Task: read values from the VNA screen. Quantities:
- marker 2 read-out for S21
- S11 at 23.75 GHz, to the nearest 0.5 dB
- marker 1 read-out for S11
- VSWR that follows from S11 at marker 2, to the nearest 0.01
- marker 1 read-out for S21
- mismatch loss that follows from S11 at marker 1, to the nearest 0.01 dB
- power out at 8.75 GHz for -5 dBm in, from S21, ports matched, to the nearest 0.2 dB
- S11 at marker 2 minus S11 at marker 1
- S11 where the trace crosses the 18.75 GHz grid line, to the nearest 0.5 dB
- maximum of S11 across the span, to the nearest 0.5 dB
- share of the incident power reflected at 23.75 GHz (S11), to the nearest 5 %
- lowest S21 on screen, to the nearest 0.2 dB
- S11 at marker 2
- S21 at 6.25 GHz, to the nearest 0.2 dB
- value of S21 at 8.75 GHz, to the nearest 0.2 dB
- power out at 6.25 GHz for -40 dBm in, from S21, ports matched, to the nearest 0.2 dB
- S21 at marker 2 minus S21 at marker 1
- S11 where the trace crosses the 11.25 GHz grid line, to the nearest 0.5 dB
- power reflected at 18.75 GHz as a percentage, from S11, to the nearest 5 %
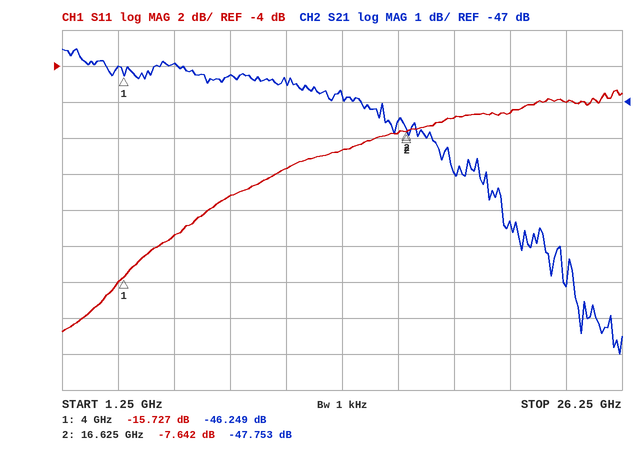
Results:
-47.753 dB
-6.0 dB
-15.727 dB
2.42
-46.249 dB
0.12 dB
-51.2 dBm
8.085 dB
-7.0 dB
-5.5 dB
25 %
-54.0 dB
-7.642 dB
-46.0 dB
-46.2 dB
-86.0 dBm
-1.504 dB
-9.5 dB
20 %
